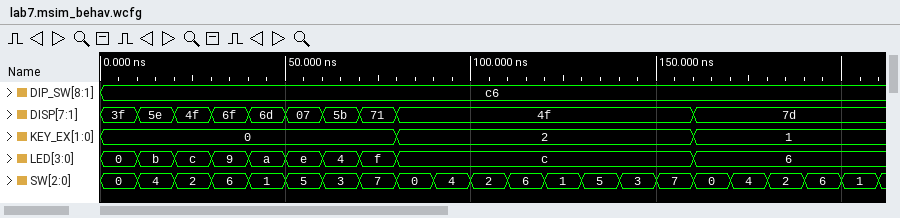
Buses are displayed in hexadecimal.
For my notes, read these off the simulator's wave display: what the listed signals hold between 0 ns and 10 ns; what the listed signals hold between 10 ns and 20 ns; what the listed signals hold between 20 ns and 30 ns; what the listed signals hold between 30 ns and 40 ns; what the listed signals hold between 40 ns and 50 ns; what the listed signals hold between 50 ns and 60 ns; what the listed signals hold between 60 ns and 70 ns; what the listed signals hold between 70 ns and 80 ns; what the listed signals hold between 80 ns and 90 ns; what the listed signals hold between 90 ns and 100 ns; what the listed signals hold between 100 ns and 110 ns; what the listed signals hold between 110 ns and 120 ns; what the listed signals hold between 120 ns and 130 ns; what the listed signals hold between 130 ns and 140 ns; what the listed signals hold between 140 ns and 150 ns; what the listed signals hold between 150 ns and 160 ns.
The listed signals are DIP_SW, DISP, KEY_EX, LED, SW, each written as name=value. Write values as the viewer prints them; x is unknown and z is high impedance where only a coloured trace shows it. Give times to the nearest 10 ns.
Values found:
DIP_SW=c6, DISP=3f, KEY_EX=0, LED=0, SW=0
DIP_SW=c6, DISP=5e, KEY_EX=0, LED=b, SW=4
DIP_SW=c6, DISP=4f, KEY_EX=0, LED=c, SW=2
DIP_SW=c6, DISP=6f, KEY_EX=0, LED=9, SW=6
DIP_SW=c6, DISP=6d, KEY_EX=0, LED=a, SW=1
DIP_SW=c6, DISP=07, KEY_EX=0, LED=e, SW=5
DIP_SW=c6, DISP=5b, KEY_EX=0, LED=4, SW=3
DIP_SW=c6, DISP=71, KEY_EX=0, LED=f, SW=7
DIP_SW=c6, DISP=4f, KEY_EX=2, LED=c, SW=0
DIP_SW=c6, DISP=4f, KEY_EX=2, LED=c, SW=4
DIP_SW=c6, DISP=4f, KEY_EX=2, LED=c, SW=2
DIP_SW=c6, DISP=4f, KEY_EX=2, LED=c, SW=6
DIP_SW=c6, DISP=4f, KEY_EX=2, LED=c, SW=1
DIP_SW=c6, DISP=4f, KEY_EX=2, LED=c, SW=5
DIP_SW=c6, DISP=4f, KEY_EX=2, LED=c, SW=3
DIP_SW=c6, DISP=4f, KEY_EX=2, LED=c, SW=7
